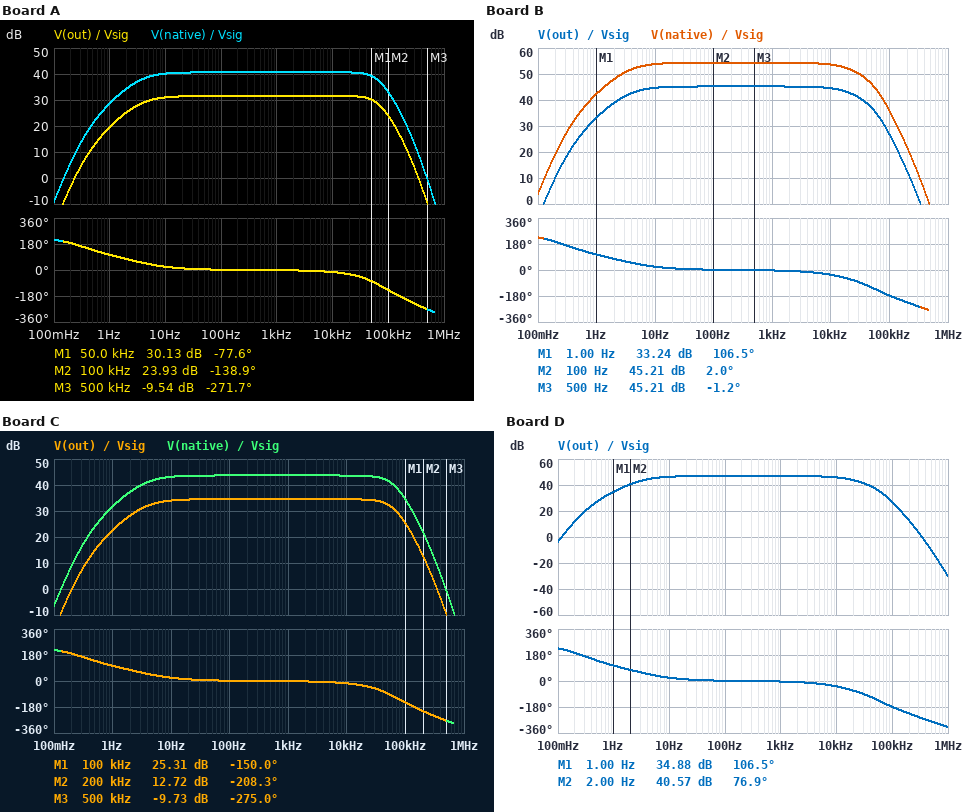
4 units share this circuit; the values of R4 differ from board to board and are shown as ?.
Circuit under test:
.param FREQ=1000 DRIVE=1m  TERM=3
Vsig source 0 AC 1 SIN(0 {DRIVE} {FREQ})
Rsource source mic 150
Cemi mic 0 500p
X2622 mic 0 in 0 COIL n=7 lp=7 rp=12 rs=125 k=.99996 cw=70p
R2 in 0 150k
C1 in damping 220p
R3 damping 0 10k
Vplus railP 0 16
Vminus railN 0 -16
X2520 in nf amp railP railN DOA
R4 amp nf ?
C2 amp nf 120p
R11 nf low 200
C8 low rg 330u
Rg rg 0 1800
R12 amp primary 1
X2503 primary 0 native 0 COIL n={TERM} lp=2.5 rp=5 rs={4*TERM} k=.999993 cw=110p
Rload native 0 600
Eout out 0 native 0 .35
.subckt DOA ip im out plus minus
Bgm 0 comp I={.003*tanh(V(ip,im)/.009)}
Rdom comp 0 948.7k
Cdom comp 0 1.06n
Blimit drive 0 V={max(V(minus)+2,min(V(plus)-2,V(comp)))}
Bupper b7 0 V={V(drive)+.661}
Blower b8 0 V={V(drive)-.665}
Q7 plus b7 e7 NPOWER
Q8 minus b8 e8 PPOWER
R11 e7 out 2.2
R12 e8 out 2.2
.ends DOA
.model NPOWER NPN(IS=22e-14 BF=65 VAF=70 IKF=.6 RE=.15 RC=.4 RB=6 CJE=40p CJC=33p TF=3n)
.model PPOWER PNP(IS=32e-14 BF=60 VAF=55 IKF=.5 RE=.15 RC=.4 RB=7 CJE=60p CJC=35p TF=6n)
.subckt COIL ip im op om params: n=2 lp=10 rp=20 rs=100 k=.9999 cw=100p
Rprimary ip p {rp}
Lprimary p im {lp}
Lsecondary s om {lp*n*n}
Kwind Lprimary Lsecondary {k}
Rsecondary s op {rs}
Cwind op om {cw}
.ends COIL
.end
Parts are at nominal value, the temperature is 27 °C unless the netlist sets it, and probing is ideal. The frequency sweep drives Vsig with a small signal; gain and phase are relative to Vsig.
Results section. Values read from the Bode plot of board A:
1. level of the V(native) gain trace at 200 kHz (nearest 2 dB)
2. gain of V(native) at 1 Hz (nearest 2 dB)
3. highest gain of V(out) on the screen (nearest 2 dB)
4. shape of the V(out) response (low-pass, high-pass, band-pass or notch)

22 dB
28 dB
32 dB
band-pass
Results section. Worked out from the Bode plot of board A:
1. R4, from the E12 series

10 kΩ
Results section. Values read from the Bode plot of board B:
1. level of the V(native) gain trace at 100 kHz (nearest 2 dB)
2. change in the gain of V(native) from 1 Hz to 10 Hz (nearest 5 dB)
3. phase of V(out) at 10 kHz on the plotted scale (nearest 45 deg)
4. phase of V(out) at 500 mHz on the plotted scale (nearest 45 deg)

36 dB
10 dB
-45 deg
135 deg
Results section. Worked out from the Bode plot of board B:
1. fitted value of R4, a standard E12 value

56 kΩ
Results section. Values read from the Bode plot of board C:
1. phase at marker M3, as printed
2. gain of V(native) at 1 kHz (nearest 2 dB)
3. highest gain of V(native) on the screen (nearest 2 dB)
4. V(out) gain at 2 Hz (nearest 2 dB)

-275.0 deg
44 dB
44 dB
28 dB
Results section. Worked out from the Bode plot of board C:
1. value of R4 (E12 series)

15 kΩ
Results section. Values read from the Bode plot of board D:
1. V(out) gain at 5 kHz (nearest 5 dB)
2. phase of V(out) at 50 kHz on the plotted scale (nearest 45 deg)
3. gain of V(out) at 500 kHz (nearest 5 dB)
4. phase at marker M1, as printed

45 dB
-135 deg
-10 dB
106.5 deg
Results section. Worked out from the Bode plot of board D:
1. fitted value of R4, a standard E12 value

68 kΩ
